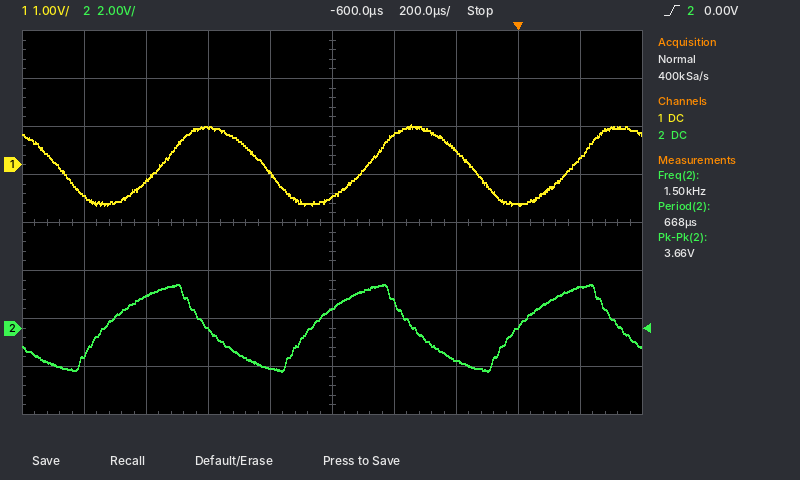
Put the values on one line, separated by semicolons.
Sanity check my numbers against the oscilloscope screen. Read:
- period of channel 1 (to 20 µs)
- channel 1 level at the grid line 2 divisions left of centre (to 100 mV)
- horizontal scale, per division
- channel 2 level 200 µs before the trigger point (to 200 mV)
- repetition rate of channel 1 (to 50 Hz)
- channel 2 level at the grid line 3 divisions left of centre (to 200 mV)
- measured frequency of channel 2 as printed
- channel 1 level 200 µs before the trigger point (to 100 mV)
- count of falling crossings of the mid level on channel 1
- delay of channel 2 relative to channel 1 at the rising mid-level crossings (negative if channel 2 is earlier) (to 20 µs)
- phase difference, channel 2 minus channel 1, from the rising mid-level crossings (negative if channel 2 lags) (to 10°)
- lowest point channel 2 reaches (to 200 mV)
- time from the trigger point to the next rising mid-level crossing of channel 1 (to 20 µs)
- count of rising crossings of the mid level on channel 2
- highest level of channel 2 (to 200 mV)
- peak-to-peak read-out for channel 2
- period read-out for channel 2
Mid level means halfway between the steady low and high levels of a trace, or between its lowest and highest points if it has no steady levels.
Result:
660 µs; 800 mV; 200 µs; -1.4 V; 1.50 kHz; 1.4 V; 1.50 kHz; 300 mV; 3; -180 µs; +100°; -1.8 V; 180 µs; 3; 1.8 V; 3.66 V; 668 µs
